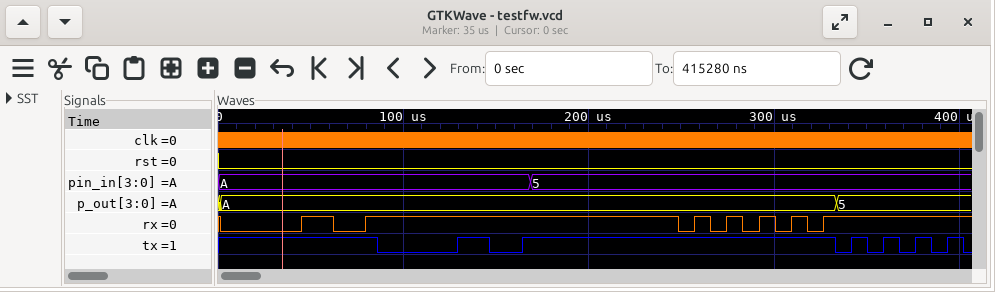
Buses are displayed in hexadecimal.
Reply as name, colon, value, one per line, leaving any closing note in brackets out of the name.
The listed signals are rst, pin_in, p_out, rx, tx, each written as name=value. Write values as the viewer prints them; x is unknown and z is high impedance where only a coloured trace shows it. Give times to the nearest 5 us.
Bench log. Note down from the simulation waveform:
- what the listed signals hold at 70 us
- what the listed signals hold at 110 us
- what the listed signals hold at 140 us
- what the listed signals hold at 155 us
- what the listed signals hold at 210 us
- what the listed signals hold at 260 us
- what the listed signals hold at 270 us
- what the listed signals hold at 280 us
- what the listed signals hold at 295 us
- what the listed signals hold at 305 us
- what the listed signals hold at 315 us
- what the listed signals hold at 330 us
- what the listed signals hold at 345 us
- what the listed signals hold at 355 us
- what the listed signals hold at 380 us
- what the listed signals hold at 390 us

what the listed signals hold at 70 us: rst=0, pin_in=A, p_out=A, rx=0, tx=1
what the listed signals hold at 110 us: rst=0, pin_in=A, p_out=A, rx=1, tx=0
what the listed signals hold at 140 us: rst=0, pin_in=A, p_out=A, rx=1, tx=1
what the listed signals hold at 155 us: rst=0, pin_in=A, p_out=A, rx=1, tx=0
what the listed signals hold at 210 us: rst=0, pin_in=5, p_out=A, rx=1, tx=1
what the listed signals hold at 260 us: rst=0, pin_in=5, p_out=A, rx=1, tx=1
what the listed signals hold at 270 us: rst=0, pin_in=5, p_out=A, rx=0, tx=1
what the listed signals hold at 280 us: rst=0, pin_in=5, p_out=A, rx=1, tx=1
what the listed signals hold at 295 us: rst=0, pin_in=5, p_out=A, rx=1, tx=1
what the listed signals hold at 305 us: rst=0, pin_in=5, p_out=A, rx=0, tx=1
what the listed signals hold at 315 us: rst=0, pin_in=5, p_out=A, rx=1, tx=1
what the listed signals hold at 330 us: rst=0, pin_in=5, p_out=A, rx=1, tx=1
what the listed signals hold at 345 us: rst=0, pin_in=5, p_out=5, rx=1, tx=1
what the listed signals hold at 355 us: rst=0, pin_in=5, p_out=5, rx=1, tx=0
what the listed signals hold at 380 us: rst=0, pin_in=5, p_out=5, rx=1, tx=1
what the listed signals hold at 390 us: rst=0, pin_in=5, p_out=5, rx=1, tx=0
